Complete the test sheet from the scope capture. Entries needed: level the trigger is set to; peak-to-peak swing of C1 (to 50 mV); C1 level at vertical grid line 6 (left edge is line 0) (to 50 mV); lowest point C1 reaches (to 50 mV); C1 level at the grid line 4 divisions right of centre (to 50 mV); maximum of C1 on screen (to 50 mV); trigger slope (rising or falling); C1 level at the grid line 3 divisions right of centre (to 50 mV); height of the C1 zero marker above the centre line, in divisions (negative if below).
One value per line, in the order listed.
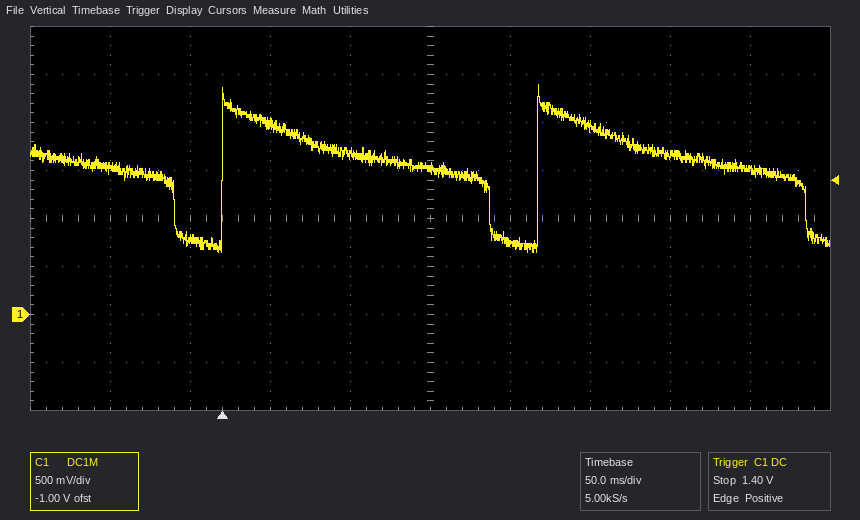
1.40 V
1.75 V
750 mV
650 mV
1.50 V
2.40 V
rising
1.65 V
-2.0 div
